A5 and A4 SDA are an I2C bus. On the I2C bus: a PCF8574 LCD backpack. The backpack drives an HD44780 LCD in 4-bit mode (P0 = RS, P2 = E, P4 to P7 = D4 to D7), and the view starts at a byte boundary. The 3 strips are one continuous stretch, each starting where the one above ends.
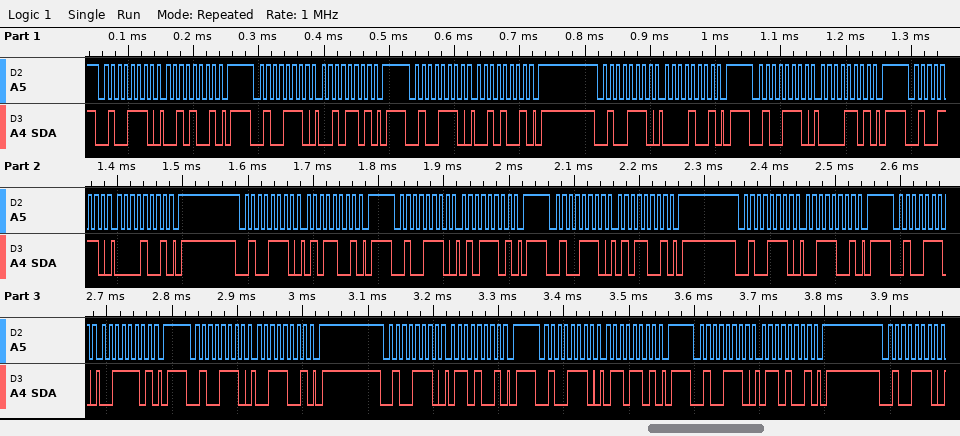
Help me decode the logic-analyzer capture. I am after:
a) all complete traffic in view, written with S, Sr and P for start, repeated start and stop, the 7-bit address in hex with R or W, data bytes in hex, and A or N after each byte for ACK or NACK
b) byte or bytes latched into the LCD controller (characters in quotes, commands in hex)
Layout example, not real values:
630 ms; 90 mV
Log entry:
S 27W A 29 A P S 27W A 2D A P S 27W A 29 A P S 27W A 09 A P S 27W A 0D A P S 27W A 09 A P S 27W A 59 A P S 27W A 5D A P S 27W A 59 A P S 27W A 39 A P S 27W A 3D A P S 27W A 39 A P S 27W A 69 A P S 27W A 6D A P S 27W A 69 A P S 27W A; ' ' 'S'
